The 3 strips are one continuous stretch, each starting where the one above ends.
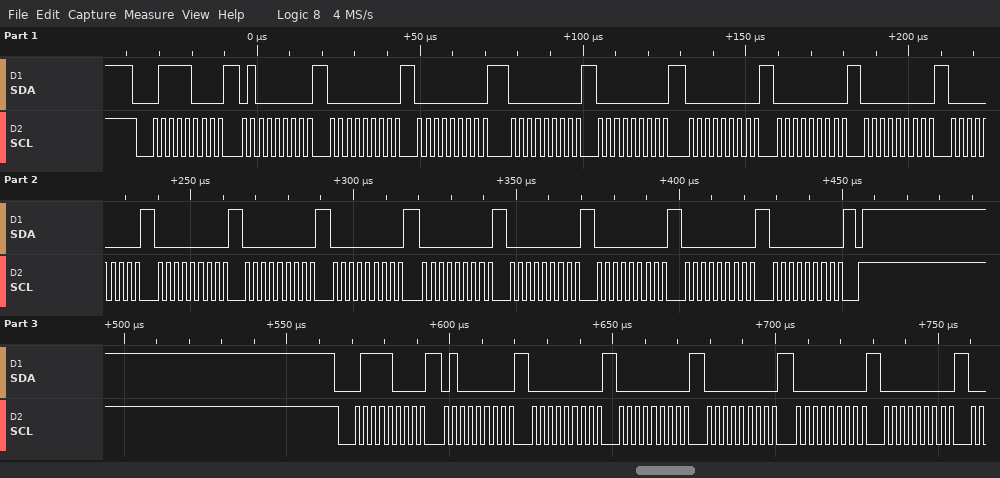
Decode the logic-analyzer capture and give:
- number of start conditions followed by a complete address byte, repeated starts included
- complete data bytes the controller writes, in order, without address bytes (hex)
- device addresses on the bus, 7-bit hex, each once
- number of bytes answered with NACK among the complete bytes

2
40 00 00 00 00 00 00 00 00 00 00 00 00 00 00 00 00 40 00 00 00 00 00
0x3C
0
